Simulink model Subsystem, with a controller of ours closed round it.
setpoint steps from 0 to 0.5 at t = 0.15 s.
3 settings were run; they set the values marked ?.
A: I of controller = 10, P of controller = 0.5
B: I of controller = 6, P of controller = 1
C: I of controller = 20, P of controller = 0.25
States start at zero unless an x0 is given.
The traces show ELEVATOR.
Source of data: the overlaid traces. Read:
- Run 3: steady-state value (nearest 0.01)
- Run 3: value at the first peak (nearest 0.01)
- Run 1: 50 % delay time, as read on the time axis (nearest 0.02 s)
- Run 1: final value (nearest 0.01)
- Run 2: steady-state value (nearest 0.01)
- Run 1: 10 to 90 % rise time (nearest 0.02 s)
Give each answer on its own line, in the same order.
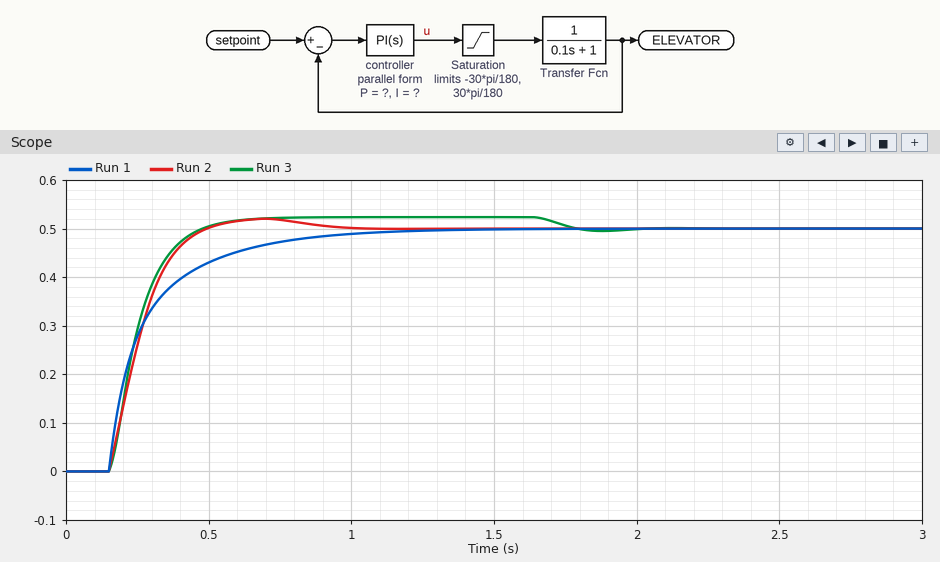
0.50
0.52
0.24 s
0.50
0.50
0.42 s
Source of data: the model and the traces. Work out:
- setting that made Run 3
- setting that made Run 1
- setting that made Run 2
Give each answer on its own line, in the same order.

C
B
A
